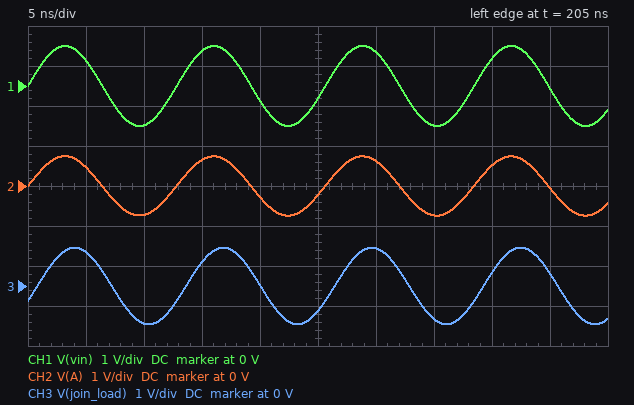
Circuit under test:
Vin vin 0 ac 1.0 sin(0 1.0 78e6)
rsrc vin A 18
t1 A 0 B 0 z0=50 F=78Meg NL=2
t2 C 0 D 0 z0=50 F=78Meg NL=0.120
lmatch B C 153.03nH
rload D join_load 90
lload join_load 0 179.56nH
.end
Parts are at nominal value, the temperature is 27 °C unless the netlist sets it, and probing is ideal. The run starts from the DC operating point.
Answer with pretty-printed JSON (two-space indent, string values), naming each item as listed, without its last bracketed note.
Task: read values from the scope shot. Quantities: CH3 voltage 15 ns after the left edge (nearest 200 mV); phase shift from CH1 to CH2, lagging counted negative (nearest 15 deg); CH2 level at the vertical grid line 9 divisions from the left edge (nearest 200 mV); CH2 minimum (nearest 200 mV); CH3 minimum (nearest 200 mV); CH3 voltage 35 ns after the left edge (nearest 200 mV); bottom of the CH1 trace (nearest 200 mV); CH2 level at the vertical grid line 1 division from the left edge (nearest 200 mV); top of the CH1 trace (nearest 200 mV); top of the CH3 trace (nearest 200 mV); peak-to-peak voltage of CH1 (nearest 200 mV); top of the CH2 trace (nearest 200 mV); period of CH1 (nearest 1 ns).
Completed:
{
  "CH3 voltage 15 ns after the left edge": "600 mV",
  "phase shift from CH1 to CH2, lagging counted negative": "0 deg",
  "CH2 level at the vertical grid line 9 divisions from the left edge": "0 V",
  "CH2 minimum": "-800 mV",
  "CH3 minimum": "-1.0 V",
  "CH3 voltage 35 ns after the left edge": "-800 mV",
  "bottom of the CH1 trace": "-1.0 V",
  "CH2 level at the vertical grid line 1 division from the left edge": "400 mV",
  "top of the CH1 trace": "1.0 V",
  "top of the CH3 trace": "1.0 V",
  "peak-to-peak voltage of CH1": "2.0 V",
  "top of the CH2 trace": "800 mV",
  "period of CH1": "13 ns"
}
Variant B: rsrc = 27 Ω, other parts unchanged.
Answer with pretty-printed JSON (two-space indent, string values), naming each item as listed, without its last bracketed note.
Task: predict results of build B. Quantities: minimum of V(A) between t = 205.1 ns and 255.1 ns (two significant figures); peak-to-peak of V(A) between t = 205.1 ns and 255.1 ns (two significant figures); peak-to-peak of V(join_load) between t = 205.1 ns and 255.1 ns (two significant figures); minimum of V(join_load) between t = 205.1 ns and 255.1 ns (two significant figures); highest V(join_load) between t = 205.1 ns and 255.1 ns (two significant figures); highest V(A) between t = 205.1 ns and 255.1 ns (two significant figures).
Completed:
{
  "minimum of V(A) between t = 205.1 ns and 255.1 ns": "-660 mV",
  "peak-to-peak of V(A) between t = 205.1 ns and 255.1 ns": "1.3 V",
  "peak-to-peak of V(join_load) between t = 205.1 ns and 255.1 ns": "1.7 V",
  "minimum of V(join_load) between t = 205.1 ns and 255.1 ns": "-850 mV",
  "highest V(join_load) between t = 205.1 ns and 255.1 ns": "850 mV",
  "highest V(A) between t = 205.1 ns and 255.1 ns": "660 mV"
}
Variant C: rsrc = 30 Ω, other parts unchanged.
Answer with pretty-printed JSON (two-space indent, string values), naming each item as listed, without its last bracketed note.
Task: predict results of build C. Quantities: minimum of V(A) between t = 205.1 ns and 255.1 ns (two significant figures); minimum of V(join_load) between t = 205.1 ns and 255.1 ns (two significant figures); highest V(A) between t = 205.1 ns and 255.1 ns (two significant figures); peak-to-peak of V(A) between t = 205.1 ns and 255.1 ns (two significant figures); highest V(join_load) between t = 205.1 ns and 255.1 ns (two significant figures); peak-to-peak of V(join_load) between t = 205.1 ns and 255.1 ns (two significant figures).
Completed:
{
  "minimum of V(A) between t = 205.1 ns and 255.1 ns": "-630 mV",
  "minimum of V(join_load) between t = 205.1 ns and 255.1 ns": "-820 mV",
  "highest V(A) between t = 205.1 ns and 255.1 ns": "630 mV",
  "peak-to-peak of V(A) between t = 205.1 ns and 255.1 ns": "1.3 V",
  "highest V(join_load) between t = 205.1 ns and 255.1 ns": "820 mV",
  "peak-to-peak of V(join_load) between t = 205.1 ns and 255.1 ns": "1.6 V"
}
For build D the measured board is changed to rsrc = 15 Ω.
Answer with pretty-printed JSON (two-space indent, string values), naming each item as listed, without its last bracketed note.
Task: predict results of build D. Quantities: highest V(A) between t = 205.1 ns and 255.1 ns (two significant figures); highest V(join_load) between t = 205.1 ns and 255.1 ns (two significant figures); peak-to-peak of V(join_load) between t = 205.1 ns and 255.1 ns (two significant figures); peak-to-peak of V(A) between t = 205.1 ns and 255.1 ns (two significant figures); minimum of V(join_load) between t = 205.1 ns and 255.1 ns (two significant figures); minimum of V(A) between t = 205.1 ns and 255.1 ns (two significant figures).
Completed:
{
  "highest V(A) between t = 205.1 ns and 255.1 ns": "780 mV",
  "highest V(join_load) between t = 205.1 ns and 255.1 ns": "1.0 V",
  "peak-to-peak of V(join_load) between t = 205.1 ns and 255.1 ns": "2.0 V",
  "peak-to-peak of V(A) between t = 205.1 ns and 255.1 ns": "1.6 V",
  "minimum of V(join_load) between t = 205.1 ns and 255.1 ns": "-1.0 V",
  "minimum of V(A) between t = 205.1 ns and 255.1 ns": "-780 mV"
}
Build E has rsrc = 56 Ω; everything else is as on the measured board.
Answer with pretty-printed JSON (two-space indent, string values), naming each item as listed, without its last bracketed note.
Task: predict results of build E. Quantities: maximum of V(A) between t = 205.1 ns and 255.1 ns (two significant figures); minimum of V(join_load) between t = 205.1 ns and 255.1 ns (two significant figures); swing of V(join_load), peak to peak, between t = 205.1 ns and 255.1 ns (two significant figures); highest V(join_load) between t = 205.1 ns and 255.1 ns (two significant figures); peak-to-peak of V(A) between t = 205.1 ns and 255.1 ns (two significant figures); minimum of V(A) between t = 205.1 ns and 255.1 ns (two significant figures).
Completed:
{
  "maximum of V(A) between t = 205.1 ns and 255.1 ns": "480 mV",
  "minimum of V(join_load) between t = 205.1 ns and 255.1 ns": "-620 mV",
  "swing of V(join_load), peak to peak, between t = 205.1 ns and 255.1 ns": "1.2 V",
  "highest V(join_load) between t = 205.1 ns and 255.1 ns": "620 mV",
  "peak-to-peak of V(A) between t = 205.1 ns and 255.1 ns": "960 mV",
  "minimum of V(A) between t = 205.1 ns and 255.1 ns": "-480 mV"
}
